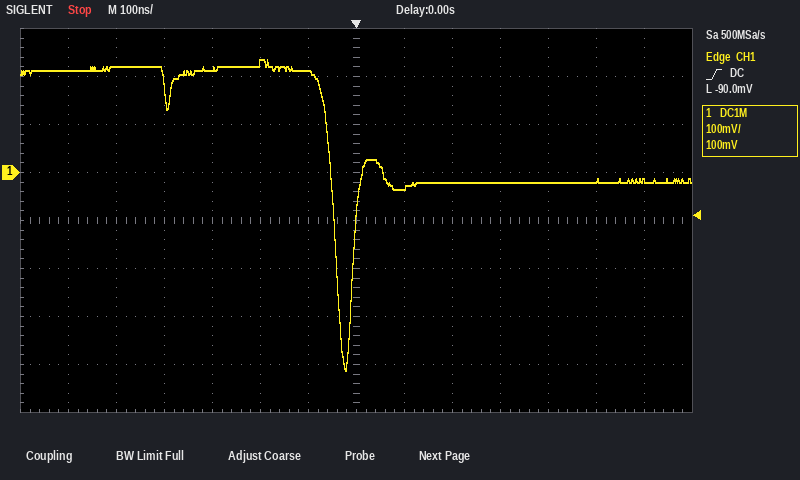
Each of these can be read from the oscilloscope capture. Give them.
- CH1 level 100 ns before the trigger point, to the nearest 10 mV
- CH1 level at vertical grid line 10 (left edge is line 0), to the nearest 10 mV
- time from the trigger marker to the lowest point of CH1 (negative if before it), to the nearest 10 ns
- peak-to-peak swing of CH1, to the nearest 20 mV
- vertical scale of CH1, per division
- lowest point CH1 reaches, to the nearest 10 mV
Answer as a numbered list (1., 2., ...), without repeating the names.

1. 210 mV
2. -20 mV
3. -20 ns
4. 640 mV
5. 100 mV
6. -410 mV
